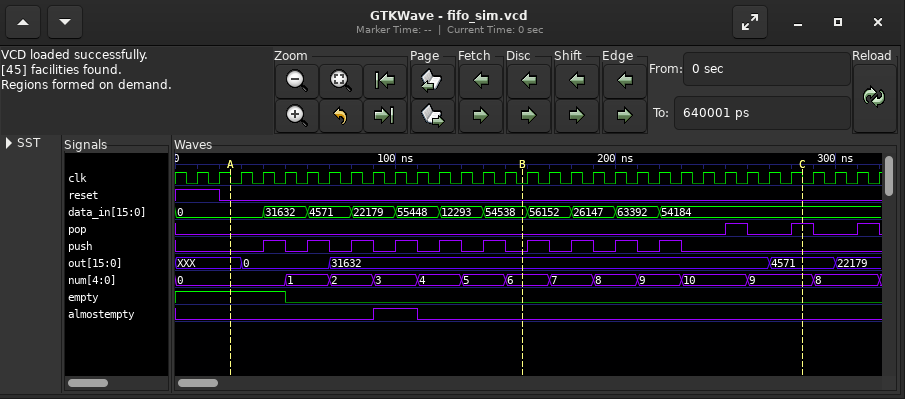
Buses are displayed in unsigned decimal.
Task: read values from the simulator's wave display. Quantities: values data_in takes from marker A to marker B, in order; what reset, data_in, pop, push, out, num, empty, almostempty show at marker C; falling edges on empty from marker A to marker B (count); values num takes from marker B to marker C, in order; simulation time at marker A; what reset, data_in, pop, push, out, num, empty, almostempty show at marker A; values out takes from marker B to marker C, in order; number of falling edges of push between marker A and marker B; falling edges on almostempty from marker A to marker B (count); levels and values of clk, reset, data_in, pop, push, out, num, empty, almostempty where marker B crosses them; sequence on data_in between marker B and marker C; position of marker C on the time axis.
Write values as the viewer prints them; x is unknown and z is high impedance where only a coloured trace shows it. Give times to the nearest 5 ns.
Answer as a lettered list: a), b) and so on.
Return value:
a) 0, 31632, 4571, 22179, 55448, 12293, 54538
b) reset=0, data_in=54184, pop=1, push=0, out=4571, num=9, empty=0, almostempty=0
c) 1
d) 6, 7, 8, 9, 10, 9
e) 25 ns
f) reset=0, data_in=0, pop=0, push=0, out=XXX, num=0, empty=1, almostempty=0
g) 31632, 4571
h) 6
i) 1
j) clk=0, reset=0, data_in=54538, pop=0, push=0, out=31632, num=6, empty=0, almostempty=0
k) 54538, 56152, 26147, 63392, 54184
l) 285 ns
